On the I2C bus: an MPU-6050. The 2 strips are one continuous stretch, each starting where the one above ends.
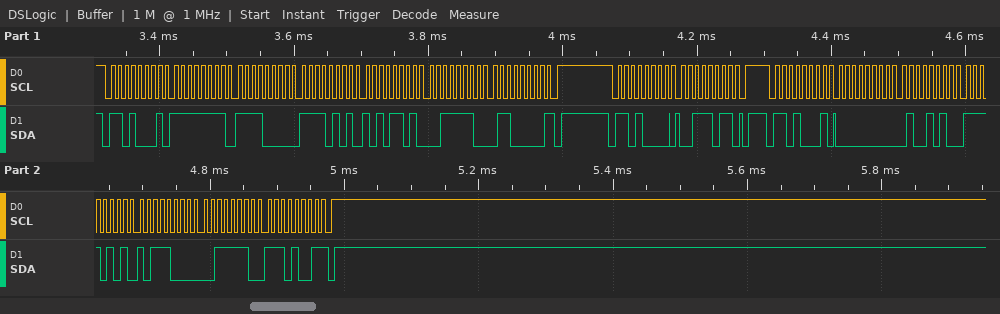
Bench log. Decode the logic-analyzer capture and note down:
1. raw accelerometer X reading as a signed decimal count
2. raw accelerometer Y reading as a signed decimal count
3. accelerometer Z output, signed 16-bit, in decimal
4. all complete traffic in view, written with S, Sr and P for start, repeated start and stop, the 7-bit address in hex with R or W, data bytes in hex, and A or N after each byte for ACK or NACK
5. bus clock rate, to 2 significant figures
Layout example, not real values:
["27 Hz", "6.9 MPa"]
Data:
["74", "-2632", "16105", "S 68R A FF A F0 A F5 A AD A 3E A 60 N P S 68W A 3B A P S 68R A 00 A 4A A F5 A B8 A 3E A E9 N P", "100 kHz"]
